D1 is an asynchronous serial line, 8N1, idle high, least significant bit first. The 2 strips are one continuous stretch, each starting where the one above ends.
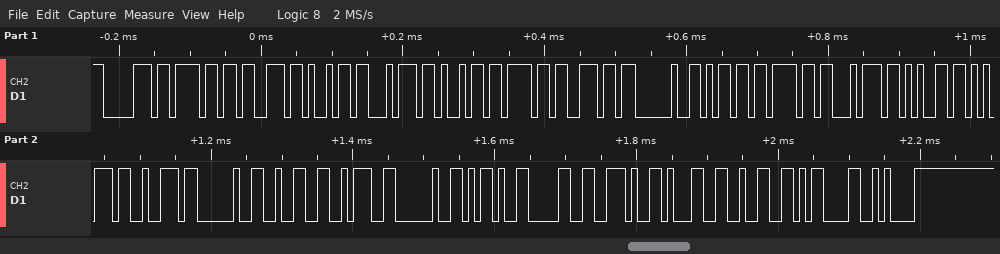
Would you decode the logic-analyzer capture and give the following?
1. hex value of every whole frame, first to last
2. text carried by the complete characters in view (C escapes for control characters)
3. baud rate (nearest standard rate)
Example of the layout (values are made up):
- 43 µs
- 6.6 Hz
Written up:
- 70 6F 73 69 74 69 6F 6E 20 6D 6F 74 65 75 72 20 32 3A 20 2D 30 2E 31 32 0D 0A
- "position moteur 2: -0.12\r\n"
- 115200 baud
